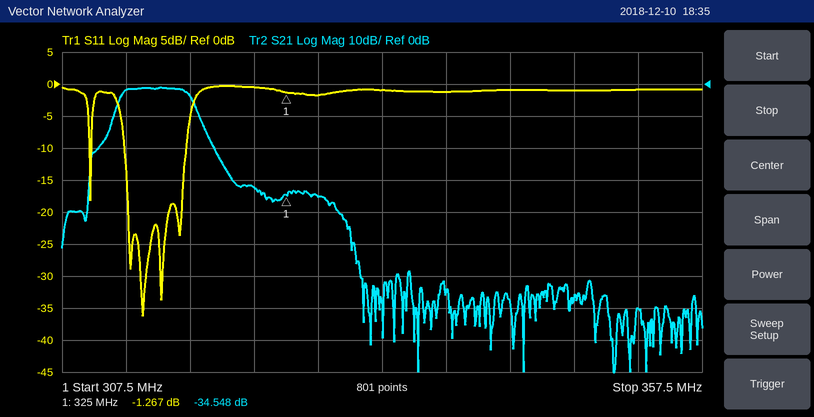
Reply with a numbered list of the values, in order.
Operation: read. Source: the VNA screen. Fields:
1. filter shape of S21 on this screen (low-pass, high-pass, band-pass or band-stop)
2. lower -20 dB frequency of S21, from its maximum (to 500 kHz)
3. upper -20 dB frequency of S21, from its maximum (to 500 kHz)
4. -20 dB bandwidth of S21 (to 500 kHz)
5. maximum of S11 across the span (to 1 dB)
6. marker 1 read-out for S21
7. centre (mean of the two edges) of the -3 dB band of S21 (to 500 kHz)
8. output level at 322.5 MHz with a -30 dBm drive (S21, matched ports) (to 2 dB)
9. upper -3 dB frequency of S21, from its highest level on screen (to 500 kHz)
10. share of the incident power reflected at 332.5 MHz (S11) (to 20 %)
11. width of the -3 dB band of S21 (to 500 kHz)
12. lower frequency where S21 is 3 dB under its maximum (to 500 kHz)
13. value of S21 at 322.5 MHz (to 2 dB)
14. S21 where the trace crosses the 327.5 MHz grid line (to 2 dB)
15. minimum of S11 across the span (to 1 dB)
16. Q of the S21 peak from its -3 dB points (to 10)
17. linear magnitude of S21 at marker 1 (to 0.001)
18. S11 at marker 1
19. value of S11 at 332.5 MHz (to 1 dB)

1. band-pass
2. 310.0 MHz
3. 319.5 MHz
4. 9.5 MHz
5. 0 dB
6. -34.548 dB
7. 315.0 MHz
8. -62 dBm
9. 317.5 MHz
10. 80 %
11. 5.5 MHz
12. 312.0 MHz
13. -32 dB
14. -36 dB
15. -36 dB
16. 60
17. 0.019
18. -1.267 dB
19. -1 dB
